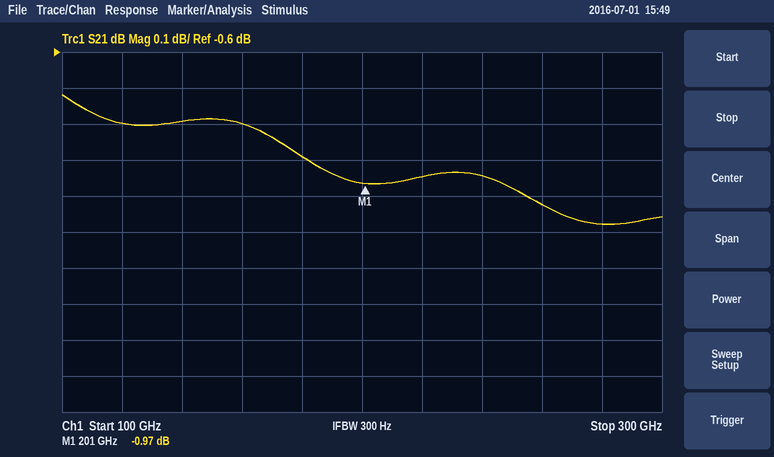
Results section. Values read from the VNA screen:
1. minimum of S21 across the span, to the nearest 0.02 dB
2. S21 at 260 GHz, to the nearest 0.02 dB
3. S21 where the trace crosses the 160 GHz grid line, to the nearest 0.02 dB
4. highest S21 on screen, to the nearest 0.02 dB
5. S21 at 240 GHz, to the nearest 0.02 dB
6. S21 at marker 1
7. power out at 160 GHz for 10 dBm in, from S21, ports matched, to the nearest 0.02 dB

-1.08 dB
-1.02 dB
-0.80 dB
-0.72 dB
-0.94 dB
-0.97 dB
9.20 dBm
